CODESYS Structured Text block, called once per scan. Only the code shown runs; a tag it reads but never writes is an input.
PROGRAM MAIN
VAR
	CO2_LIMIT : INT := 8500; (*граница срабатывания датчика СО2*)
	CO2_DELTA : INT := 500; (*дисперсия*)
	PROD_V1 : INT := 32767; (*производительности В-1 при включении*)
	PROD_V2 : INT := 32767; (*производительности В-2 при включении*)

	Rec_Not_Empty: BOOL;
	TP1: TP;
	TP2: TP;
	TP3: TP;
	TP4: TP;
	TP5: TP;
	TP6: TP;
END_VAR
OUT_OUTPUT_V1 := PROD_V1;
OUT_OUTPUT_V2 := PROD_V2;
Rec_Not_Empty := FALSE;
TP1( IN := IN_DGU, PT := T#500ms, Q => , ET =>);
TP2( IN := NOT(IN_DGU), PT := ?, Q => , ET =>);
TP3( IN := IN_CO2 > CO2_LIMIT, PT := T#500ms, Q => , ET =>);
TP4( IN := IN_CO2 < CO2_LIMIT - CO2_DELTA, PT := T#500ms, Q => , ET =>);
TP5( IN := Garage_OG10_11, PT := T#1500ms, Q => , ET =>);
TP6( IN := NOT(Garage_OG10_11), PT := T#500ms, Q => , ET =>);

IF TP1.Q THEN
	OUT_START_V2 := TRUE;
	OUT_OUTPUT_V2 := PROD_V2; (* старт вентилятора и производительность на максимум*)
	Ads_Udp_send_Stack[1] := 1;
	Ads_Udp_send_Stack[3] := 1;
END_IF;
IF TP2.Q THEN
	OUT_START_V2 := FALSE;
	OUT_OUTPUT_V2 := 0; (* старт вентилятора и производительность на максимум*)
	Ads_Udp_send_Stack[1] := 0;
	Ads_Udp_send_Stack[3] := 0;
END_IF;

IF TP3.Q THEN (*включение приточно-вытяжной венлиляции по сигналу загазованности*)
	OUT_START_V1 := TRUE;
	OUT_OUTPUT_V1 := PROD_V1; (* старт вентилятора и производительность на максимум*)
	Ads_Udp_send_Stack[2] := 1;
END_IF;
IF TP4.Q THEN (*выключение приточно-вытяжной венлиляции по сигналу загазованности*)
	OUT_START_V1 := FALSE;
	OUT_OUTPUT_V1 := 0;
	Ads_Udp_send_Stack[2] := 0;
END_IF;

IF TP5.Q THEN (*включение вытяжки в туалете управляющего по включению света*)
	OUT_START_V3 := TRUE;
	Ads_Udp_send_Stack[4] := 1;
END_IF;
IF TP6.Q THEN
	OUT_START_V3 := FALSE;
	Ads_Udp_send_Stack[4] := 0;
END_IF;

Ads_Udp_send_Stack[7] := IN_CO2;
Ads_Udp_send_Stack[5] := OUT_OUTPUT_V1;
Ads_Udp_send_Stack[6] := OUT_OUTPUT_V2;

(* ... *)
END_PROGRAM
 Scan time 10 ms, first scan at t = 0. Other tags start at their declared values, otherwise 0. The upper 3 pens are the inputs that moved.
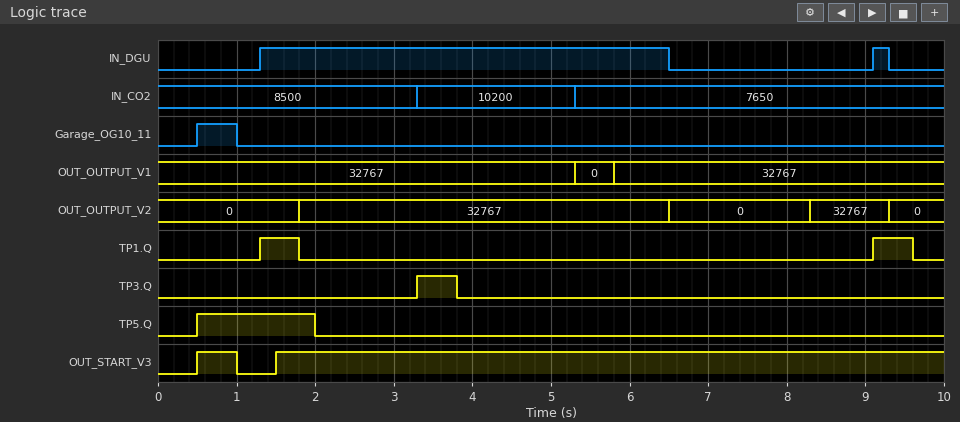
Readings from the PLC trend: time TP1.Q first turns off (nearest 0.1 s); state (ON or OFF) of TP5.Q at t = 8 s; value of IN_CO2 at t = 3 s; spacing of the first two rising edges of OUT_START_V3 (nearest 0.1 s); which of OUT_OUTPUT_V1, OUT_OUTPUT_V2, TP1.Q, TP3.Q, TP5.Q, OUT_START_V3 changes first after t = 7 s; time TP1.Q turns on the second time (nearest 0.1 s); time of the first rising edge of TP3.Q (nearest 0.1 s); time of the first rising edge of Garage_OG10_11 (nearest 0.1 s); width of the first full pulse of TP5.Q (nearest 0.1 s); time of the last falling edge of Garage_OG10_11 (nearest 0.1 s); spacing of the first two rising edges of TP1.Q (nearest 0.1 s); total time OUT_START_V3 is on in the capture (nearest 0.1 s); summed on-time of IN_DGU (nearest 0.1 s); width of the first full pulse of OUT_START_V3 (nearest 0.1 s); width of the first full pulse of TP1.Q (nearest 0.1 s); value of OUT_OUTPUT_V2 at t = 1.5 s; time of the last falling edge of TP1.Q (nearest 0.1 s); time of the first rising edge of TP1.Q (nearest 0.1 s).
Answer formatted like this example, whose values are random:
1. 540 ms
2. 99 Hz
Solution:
1. 1.8 s
2. OFF
3. 8500
4. 1.0 s
5. OUT_OUTPUT_V2
6. 9.1 s
7. 3.3 s
8. 0.5 s
9. 1.5 s
10. 1.0 s
11. 7.8 s
12. 9.0 s
13. 5.4 s
14. 0.5 s
15. 0.5 s
16. 0
17. 9.6 s
18. 1.3 s
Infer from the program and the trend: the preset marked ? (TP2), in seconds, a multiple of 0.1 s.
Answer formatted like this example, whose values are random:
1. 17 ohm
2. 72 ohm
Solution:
1. 1.8 s
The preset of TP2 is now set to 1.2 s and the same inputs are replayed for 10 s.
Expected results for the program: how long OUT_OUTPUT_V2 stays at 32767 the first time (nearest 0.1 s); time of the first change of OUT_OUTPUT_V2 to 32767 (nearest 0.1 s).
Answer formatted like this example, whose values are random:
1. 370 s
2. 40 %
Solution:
1. 5.3 s
2. 1.2 s
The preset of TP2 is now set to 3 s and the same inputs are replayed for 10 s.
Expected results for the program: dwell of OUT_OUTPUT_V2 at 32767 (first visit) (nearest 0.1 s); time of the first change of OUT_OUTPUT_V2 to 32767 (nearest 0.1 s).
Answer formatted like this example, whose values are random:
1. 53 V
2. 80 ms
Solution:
1. 3.5 s
2. 3.0 s
